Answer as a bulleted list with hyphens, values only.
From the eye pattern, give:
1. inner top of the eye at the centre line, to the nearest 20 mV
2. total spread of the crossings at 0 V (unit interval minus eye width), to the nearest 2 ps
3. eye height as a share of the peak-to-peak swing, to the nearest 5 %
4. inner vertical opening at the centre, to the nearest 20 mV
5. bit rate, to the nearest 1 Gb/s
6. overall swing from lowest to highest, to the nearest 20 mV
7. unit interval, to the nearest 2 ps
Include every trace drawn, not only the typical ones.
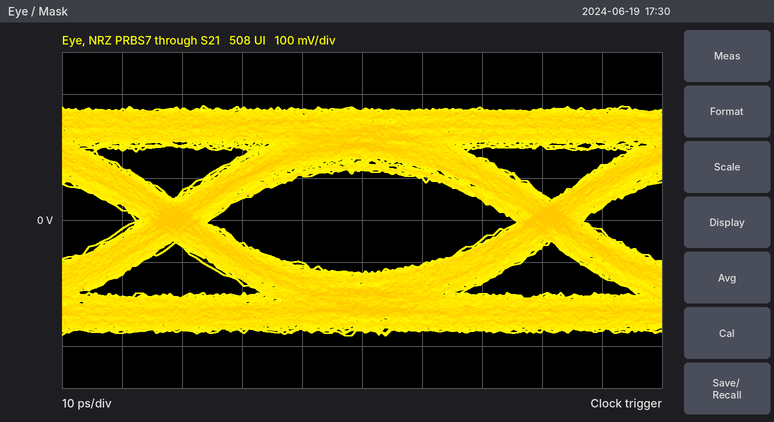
- 120 mV
- 12 ps
- 45 %
- 240 mV
- 16 Gb/s
- 540 mV
- 62 ps
